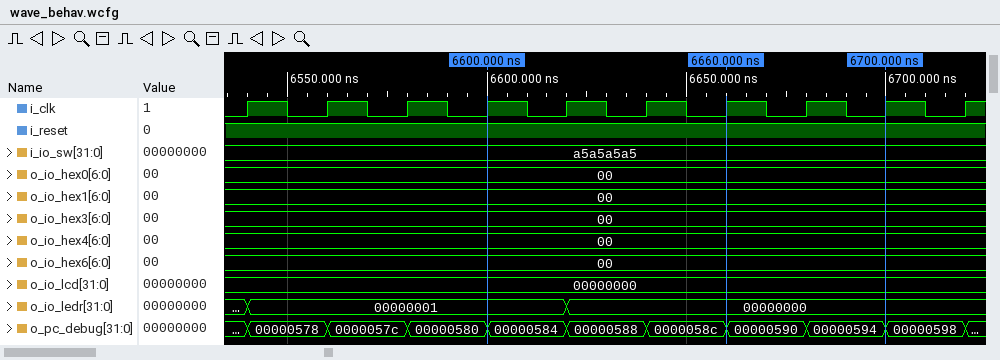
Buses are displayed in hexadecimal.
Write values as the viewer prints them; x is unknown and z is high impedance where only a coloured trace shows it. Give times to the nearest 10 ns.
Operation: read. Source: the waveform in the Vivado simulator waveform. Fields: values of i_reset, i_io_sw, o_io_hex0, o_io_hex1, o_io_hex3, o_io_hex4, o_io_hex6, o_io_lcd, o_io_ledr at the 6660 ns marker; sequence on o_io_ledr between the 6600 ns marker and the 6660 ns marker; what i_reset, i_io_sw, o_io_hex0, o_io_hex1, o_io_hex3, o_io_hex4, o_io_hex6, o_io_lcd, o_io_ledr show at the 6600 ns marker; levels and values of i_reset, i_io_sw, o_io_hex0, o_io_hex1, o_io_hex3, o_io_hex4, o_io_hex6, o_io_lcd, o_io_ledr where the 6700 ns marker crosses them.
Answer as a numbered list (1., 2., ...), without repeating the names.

1. i_reset=1, i_io_sw=a5a5a5a5, o_io_hex0=00, o_io_hex1=00, o_io_hex3=00, o_io_hex4=00, o_io_hex6=00, o_io_lcd=00000000, o_io_ledr=00000000
2. 00000001, 00000000
3. i_reset=1, i_io_sw=a5a5a5a5, o_io_hex0=00, o_io_hex1=00, o_io_hex3=00, o_io_hex4=00, o_io_hex6=00, o_io_lcd=00000000, o_io_ledr=00000001
4. i_reset=1, i_io_sw=a5a5a5a5, o_io_hex0=00, o_io_hex1=00, o_io_hex3=00, o_io_hex4=00, o_io_hex6=00, o_io_lcd=00000000, o_io_ledr=00000000
